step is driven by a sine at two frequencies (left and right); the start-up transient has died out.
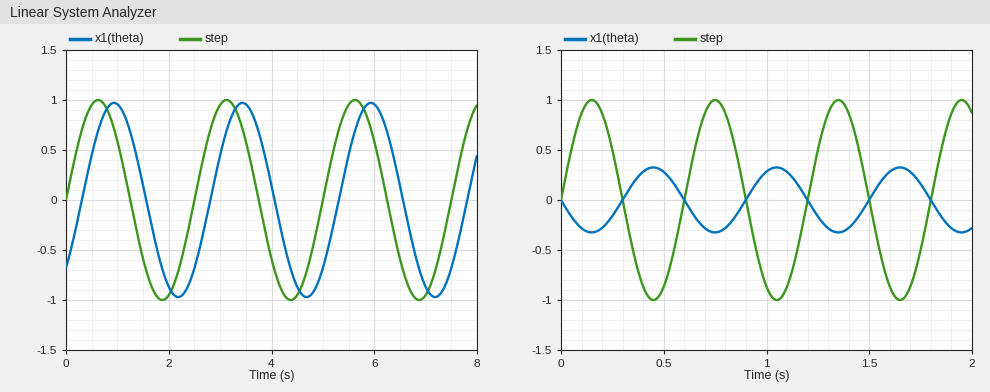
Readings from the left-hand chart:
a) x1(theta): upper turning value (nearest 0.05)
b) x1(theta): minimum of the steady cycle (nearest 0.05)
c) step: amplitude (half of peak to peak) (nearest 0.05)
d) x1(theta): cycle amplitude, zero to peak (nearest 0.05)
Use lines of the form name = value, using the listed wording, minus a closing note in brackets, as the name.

x1(theta): upper turning value = 0.95
x1(theta): minimum of the steady cycle = -0.95
step: amplitude (half of peak to peak) = 1.00
x1(theta): cycle amplitude, zero to peak = 0.95
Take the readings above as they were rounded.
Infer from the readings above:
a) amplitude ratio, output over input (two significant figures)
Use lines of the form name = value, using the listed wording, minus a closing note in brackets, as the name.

amplitude ratio, output over input = 0.95
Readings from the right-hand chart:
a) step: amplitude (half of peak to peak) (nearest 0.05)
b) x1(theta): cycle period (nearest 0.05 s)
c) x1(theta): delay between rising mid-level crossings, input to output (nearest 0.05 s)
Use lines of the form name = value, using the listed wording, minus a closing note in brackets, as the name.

step: amplitude (half of peak to peak) = 1.00
x1(theta): cycle period = 0.60 s
x1(theta): delay between rising mid-level crossings, input to output = 0.30 s
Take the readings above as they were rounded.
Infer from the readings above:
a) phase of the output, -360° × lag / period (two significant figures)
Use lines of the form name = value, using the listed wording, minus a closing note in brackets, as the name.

phase of the output, -360° × lag / period = -180°
